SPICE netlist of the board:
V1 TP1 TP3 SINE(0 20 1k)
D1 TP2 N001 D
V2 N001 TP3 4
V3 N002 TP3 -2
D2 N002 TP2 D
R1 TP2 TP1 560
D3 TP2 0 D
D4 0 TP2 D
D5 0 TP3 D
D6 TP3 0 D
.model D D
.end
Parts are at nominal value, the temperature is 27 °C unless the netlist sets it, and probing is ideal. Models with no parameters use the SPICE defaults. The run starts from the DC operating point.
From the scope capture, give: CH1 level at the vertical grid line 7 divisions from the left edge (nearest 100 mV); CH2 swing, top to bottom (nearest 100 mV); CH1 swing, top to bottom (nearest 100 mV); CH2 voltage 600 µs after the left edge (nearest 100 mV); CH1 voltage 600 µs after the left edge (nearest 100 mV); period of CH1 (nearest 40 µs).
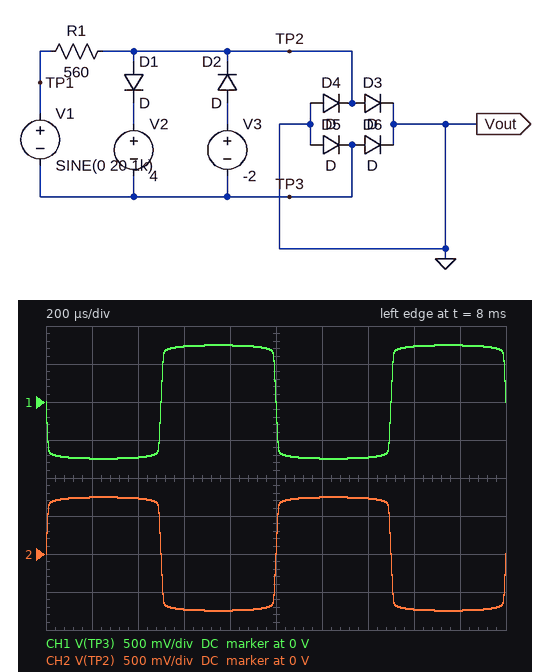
-700 mV
1.5 V
1.5 V
-700 mV
700 mV
1.00 ms
